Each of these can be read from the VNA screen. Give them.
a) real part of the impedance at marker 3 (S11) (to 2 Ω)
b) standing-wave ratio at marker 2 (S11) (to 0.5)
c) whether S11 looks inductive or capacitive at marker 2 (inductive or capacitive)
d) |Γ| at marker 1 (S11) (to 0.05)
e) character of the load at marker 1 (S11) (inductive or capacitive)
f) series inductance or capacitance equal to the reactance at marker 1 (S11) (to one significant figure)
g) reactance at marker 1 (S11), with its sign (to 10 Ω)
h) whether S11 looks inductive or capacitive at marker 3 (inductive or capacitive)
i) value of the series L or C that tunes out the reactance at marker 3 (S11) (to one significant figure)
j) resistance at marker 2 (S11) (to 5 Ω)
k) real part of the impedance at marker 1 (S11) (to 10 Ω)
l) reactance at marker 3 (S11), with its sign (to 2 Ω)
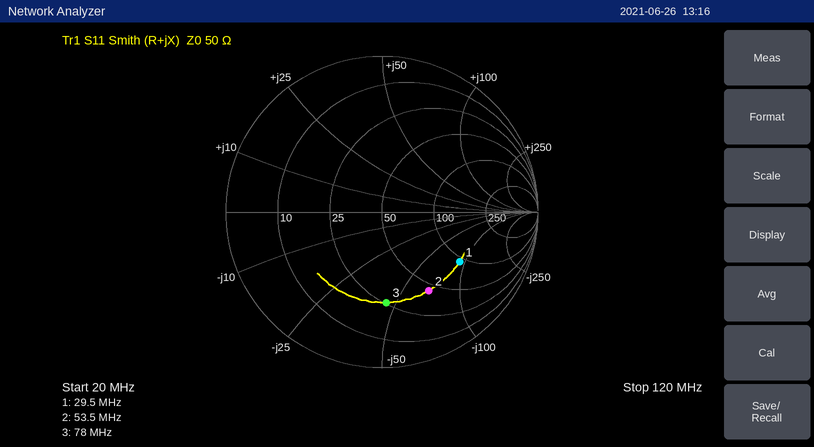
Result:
26 Ω
4.0
capacitive
0.60
capacitive
60 pF
-90 Ω
capacitive
90 nH
45 Ω
90 Ω
-46 Ω
